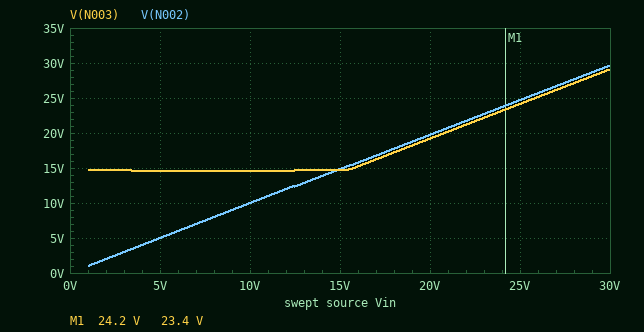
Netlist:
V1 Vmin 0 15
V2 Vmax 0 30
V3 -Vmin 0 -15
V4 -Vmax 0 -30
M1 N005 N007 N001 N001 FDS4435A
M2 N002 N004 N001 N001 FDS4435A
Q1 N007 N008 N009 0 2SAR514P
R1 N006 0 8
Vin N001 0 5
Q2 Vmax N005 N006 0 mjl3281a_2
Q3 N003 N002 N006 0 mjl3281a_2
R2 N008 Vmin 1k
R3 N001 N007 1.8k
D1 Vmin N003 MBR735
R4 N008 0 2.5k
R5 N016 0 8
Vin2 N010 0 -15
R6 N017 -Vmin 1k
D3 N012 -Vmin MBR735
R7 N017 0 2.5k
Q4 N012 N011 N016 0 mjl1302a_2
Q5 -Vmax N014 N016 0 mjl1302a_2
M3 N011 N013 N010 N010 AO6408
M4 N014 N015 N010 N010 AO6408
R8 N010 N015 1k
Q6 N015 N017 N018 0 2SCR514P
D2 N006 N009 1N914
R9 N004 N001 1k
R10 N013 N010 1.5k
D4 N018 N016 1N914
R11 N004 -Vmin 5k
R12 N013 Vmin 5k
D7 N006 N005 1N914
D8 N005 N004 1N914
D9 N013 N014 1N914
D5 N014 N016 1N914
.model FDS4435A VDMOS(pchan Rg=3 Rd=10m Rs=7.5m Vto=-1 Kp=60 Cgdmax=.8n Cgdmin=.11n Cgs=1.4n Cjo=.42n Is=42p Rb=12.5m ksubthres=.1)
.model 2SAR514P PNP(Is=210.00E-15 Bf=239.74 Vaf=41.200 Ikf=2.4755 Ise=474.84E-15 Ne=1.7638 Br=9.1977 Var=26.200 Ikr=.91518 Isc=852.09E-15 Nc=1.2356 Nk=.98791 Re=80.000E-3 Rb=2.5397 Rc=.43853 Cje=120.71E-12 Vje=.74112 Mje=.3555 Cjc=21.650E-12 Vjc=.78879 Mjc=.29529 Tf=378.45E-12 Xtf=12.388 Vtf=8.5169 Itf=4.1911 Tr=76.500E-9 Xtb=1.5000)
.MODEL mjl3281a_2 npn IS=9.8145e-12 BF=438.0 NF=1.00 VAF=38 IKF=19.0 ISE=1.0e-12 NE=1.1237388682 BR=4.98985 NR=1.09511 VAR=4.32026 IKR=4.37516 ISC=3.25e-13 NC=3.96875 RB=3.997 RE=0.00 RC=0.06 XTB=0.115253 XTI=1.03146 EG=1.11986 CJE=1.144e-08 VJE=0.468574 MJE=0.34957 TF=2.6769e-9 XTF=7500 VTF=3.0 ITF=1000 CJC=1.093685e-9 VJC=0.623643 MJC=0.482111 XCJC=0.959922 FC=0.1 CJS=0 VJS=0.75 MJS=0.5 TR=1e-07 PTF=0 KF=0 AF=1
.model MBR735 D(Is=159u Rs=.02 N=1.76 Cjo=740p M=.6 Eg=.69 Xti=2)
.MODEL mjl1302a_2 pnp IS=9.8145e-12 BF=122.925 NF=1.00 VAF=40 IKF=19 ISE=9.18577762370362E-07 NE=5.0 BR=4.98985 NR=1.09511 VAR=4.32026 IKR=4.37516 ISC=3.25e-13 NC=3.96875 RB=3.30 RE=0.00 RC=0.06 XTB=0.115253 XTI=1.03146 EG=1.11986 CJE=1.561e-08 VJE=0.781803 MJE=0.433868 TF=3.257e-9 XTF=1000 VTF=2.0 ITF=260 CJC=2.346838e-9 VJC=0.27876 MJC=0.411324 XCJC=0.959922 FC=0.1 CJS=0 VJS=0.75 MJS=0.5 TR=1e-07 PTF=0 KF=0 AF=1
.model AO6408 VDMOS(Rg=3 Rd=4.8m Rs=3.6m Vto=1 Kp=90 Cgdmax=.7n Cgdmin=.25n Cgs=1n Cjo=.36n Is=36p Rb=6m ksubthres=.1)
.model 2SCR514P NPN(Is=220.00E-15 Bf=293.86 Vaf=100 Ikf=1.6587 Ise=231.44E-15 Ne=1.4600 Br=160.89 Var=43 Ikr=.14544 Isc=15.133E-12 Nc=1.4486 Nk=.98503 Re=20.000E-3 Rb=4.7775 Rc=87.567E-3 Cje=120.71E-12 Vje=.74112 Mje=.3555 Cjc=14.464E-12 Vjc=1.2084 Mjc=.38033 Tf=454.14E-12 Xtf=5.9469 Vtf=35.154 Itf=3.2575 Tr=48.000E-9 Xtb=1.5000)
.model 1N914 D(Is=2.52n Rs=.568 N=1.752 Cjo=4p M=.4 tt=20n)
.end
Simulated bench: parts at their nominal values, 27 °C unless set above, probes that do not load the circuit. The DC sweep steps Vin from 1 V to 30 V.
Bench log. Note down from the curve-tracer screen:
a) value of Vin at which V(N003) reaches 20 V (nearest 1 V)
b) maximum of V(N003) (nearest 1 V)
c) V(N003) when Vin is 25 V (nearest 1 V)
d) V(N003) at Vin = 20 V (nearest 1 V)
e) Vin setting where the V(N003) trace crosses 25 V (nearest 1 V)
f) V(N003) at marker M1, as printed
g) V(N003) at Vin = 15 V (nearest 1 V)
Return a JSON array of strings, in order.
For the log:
["21 V", "29 V", "24 V", "19 V", "26 V", "23.4 V", "15 V"]
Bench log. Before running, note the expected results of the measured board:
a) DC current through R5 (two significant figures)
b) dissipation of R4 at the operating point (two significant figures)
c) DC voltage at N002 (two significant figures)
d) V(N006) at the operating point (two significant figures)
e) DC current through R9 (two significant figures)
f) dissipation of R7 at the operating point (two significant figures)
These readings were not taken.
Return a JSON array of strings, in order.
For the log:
["1.8 A", "46 mW", "5.0 V", "4.3 V", "1.9 mA", "67 mW"]
